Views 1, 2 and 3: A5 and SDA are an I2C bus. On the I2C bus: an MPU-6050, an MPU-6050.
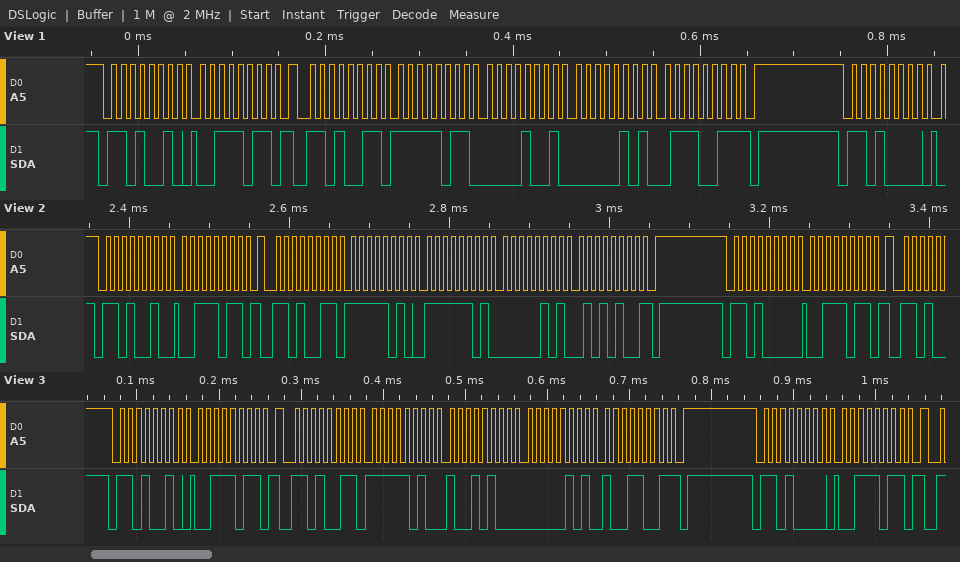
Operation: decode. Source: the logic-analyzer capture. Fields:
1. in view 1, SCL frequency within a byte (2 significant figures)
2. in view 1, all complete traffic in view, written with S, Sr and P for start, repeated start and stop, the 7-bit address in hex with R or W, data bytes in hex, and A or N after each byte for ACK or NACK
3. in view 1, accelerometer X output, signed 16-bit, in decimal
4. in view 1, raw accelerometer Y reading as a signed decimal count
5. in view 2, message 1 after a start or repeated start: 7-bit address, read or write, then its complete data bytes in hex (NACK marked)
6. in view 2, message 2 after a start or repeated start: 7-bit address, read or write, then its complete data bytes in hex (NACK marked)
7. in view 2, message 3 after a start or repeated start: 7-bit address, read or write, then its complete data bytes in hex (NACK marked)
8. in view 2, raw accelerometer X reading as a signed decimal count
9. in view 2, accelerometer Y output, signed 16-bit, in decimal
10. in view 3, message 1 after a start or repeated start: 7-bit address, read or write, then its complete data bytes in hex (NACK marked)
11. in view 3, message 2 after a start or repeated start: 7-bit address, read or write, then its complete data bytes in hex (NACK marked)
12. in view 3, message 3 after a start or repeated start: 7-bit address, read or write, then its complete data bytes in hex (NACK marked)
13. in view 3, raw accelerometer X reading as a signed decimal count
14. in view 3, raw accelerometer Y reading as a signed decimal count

100 kHz
S 69W A 3B A Sr 69R A FB A 09 A 05 A 73 N P S 68W A
-1271
1395
0x69 write: 3B
0x69 read: FA FD 05 54 NACK
0x68 write: 3B
-1283
1364
0x69 write: 3B
0x69 read: FA 94 05 99 NACK
0x68 write: 3B
-1388
1433
